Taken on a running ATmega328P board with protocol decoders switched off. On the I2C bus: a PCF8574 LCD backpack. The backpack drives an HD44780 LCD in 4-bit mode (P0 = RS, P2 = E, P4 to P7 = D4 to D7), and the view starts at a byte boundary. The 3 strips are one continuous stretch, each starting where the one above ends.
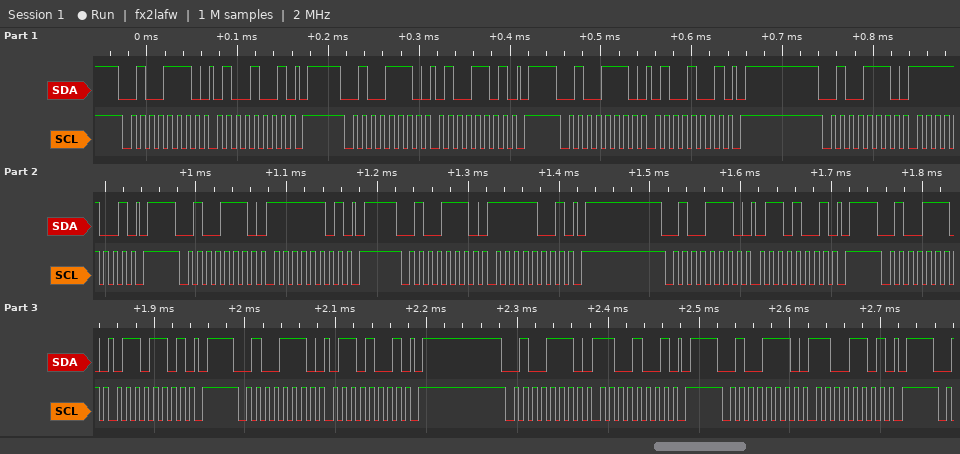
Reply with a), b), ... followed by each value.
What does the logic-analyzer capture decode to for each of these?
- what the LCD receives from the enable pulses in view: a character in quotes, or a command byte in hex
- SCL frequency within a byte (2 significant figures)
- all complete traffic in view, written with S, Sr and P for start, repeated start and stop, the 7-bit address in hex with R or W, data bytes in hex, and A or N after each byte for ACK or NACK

a) 'O'
b) 100 kHz
c) S 27W A 49 A P S 27W A 4D A P S 27W A 49 A P S 27W A F9 A P S 27W A FD A P S 27W A F9 A P S 27W A 69 A P S 27W A 6D A P S 27W A 69 A P S 27W A C9 A P S 27W A CD A P
